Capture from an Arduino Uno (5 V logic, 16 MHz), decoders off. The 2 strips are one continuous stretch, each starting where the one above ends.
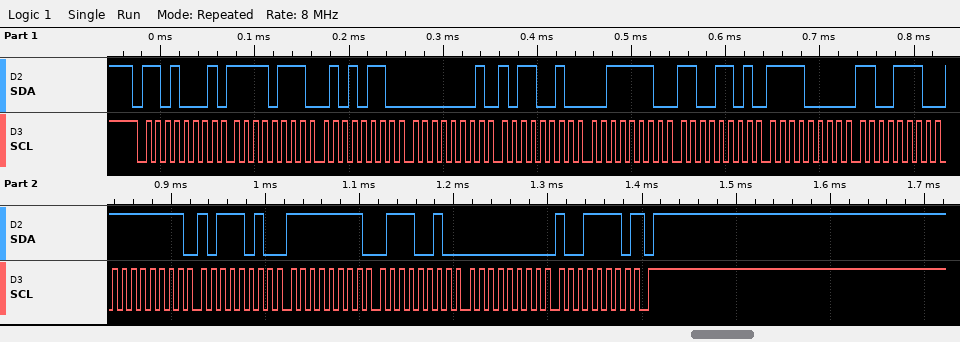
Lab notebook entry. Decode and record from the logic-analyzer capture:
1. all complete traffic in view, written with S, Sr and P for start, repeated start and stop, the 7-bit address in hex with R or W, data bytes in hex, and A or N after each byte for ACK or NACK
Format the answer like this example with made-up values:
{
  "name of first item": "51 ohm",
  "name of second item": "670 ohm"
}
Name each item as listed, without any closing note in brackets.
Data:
{
  "all complete traffic in view, written with S, Sr and P for start, repeated start and stop, the 7-bit address in hex with R or W, data bytes in hex, and A or N after each byte for ACK or NACK": "S 68R A F7 A 56 A 01 A B2 A 3E A CD A F0 A CE A FF A BA A FF A 72 A 00 A 9E N P"
}
